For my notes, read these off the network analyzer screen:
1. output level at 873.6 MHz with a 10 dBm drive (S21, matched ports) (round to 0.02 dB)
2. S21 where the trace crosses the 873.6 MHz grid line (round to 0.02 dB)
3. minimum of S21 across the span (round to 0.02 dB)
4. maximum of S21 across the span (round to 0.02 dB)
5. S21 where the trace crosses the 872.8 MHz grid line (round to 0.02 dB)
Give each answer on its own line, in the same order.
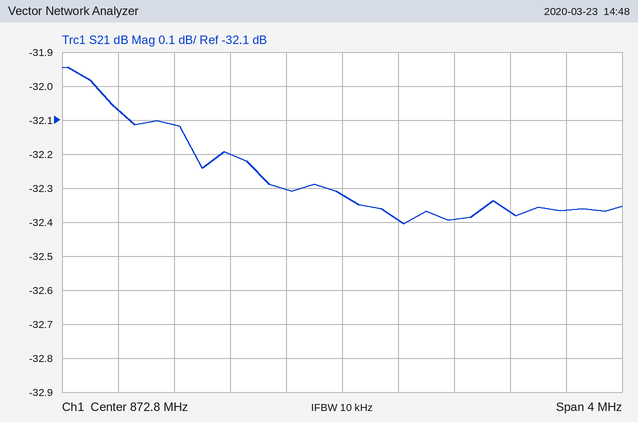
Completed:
-22.40 dBm
-32.40 dB
-32.40 dB
-31.94 dB
-32.32 dB
